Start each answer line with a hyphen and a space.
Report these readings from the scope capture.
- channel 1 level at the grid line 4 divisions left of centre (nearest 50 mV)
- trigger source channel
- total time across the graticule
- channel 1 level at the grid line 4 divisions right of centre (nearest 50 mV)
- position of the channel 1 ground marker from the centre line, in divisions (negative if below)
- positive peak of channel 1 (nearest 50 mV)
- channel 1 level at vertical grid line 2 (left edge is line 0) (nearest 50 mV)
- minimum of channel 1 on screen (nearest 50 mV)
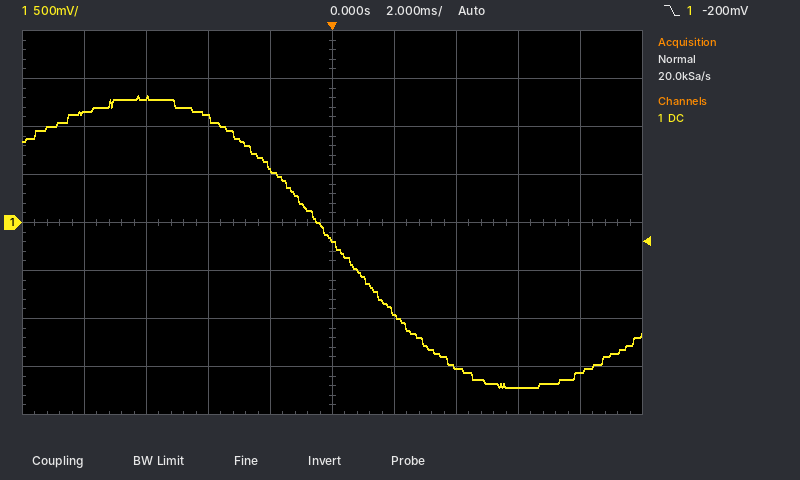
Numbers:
- 1.15 V
- channel 1
- 20 ms
- -1.55 V
- 0.0 div
- 1.30 V
- 1.30 V
- -1.70 V
